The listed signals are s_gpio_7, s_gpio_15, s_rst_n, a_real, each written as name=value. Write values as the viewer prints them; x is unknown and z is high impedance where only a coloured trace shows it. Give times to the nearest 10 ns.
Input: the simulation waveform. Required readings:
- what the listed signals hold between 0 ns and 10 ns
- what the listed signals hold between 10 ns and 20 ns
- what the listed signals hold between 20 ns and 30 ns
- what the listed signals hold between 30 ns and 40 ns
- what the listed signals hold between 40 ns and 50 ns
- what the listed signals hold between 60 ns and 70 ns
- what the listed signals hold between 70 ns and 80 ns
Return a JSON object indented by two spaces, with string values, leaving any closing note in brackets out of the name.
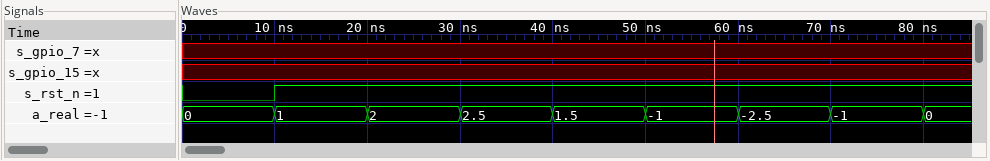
{
  "what the listed signals hold between 0 ns and 10 ns": "s_gpio_7=x, s_gpio_15=x, s_rst_n=0, a_real=0",
  "what the listed signals hold between 10 ns and 20 ns": "s_gpio_7=x, s_gpio_15=x, s_rst_n=1, a_real=1",
  "what the listed signals hold between 20 ns and 30 ns": "s_gpio_7=x, s_gpio_15=x, s_rst_n=1, a_real=2",
  "what the listed signals hold between 30 ns and 40 ns": "s_gpio_7=x, s_gpio_15=x, s_rst_n=1, a_real=2.5",
  "what the listed signals hold between 40 ns and 50 ns": "s_gpio_7=x, s_gpio_15=x, s_rst_n=1, a_real=1.5",
  "what the listed signals hold between 60 ns and 70 ns": "s_gpio_7=x, s_gpio_15=x, s_rst_n=1, a_real=-2.5",
  "what the listed signals hold between 70 ns and 80 ns": "s_gpio_7=x, s_gpio_15=x, s_rst_n=1, a_real=-1"
}
